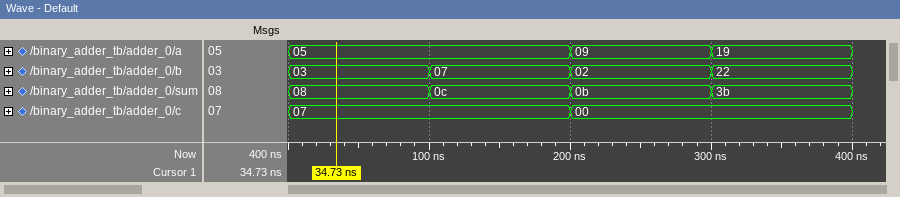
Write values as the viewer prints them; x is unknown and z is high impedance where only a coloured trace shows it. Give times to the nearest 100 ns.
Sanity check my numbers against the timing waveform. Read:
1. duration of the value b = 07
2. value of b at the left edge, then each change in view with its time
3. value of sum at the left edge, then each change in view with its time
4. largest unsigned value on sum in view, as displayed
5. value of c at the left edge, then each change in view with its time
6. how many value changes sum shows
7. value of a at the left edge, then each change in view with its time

100 ns
03, 07 at 100 ns, 02 at 200 ns, 22 at 300 ns
08, 0c at 100 ns, 0b at 200 ns, 3b at 300 ns
3b
07, 00 at 200 ns
3
05, 09 at 200 ns, 19 at 300 ns
